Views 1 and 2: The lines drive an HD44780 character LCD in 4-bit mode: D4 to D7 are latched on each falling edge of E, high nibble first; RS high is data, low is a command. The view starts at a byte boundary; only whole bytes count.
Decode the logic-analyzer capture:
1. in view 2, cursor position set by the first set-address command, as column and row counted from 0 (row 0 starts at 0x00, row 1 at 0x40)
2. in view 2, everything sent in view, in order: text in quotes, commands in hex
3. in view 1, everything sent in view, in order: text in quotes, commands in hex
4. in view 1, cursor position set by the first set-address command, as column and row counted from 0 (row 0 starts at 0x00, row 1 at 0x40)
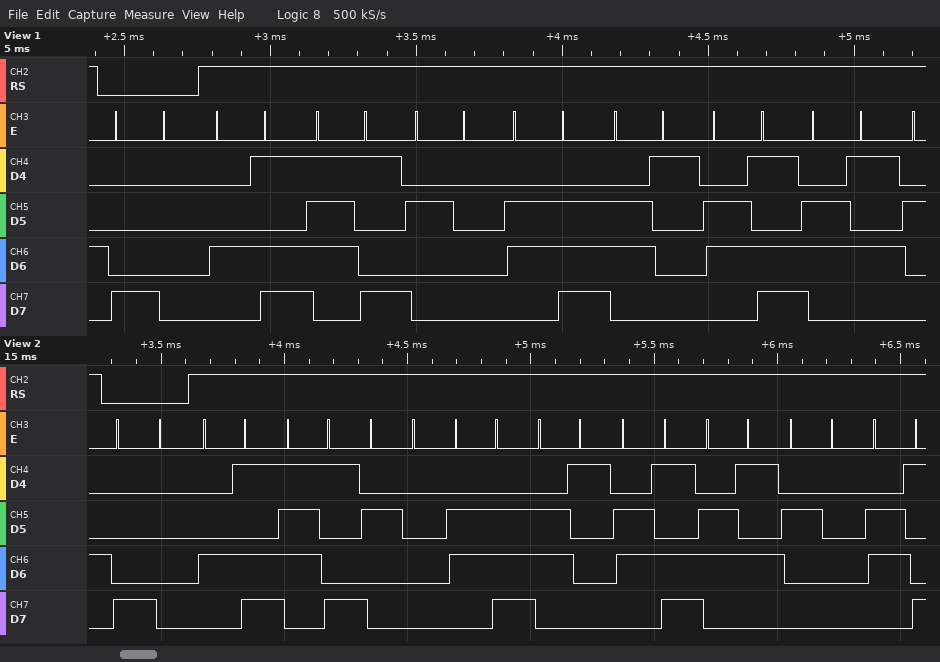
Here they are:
column 0, row 0
0x80 "My name i"
0x80 "My name"
column 0, row 0
